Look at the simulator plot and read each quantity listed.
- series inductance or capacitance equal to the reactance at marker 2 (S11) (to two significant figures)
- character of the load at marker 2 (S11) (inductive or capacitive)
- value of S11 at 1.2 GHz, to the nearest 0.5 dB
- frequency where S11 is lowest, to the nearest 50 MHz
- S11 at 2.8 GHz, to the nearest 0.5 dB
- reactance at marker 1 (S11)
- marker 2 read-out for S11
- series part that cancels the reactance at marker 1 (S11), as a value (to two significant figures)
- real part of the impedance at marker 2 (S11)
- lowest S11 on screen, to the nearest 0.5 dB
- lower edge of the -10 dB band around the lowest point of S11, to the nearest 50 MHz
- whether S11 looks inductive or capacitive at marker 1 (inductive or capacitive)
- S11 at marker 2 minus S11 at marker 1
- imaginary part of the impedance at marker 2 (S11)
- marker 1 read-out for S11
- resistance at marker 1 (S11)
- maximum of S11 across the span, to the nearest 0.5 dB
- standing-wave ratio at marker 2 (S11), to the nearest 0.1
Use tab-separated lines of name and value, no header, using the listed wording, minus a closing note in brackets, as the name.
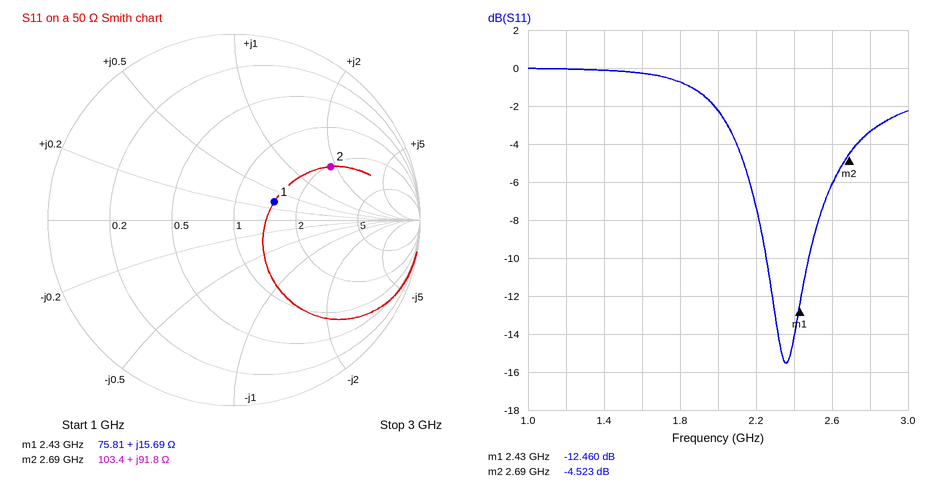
series inductance or capacitance equal to the reactance at marker 2 (S11)	5.4 nH
character of the load at marker 2 (S11)	inductive
value of S11 at 1.2 GHz, to the nearest 0.5 dB	0.0 dB
frequency where S11 is lowest, to the nearest 50 MHz	2.35 GHz
S11 at 2.8 GHz, to the nearest 0.5 dB	-3.5 dB
reactance at marker 1	+15.69 Ω
marker 2 read-out for S11	-4.523 dB
series part that cancels the reactance at marker 1 (S11), as a value	4.2 pF
real part of the impedance at marker 2	103.4 Ω
lowest S11 on screen, to the nearest 0.5 dB	-15.5 dB
lower edge of the -10 dB band around the lowest point of S11, to the nearest 50 MHz	2.25 GHz
whether S11 looks inductive or capacitive at marker 1	inductive
S11 at marker 2 minus S11 at marker 1	7.937 dB
imaginary part of the impedance at marker 2	+91.8 Ω
marker 1 read-out for S11	-12.460 dB
resistance at marker 1	75.81 Ω
maximum of S11 across the span, to the nearest 0.5 dB	0.0 dB
standing-wave ratio at marker 2 (S11), to the nearest 0.1	3.9
